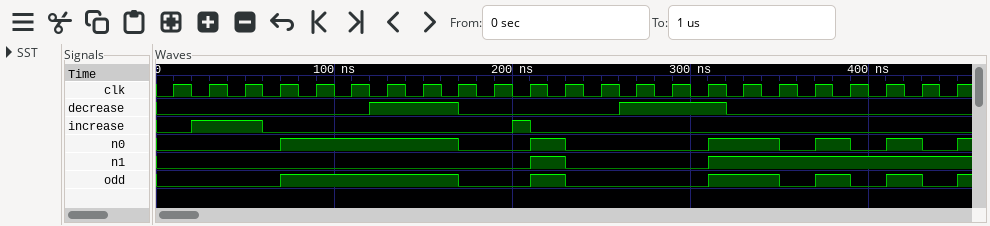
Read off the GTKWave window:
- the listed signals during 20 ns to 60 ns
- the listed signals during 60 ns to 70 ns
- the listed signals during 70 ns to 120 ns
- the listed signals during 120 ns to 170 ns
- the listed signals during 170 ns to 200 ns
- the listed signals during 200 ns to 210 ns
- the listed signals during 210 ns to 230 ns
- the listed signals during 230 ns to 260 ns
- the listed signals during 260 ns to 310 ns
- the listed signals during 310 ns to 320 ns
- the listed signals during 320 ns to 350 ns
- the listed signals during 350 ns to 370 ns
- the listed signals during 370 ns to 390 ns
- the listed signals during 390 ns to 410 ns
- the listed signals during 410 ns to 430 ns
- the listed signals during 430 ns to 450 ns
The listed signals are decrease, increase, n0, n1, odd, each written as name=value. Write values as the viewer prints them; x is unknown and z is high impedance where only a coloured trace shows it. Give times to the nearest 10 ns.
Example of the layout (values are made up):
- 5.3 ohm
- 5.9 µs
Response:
- decrease=0, increase=1, n0=0, n1=0, odd=0
- decrease=0, increase=0, n0=0, n1=0, odd=0
- decrease=0, increase=0, n0=1, n1=0, odd=1
- decrease=1, increase=0, n0=1, n1=0, odd=1
- decrease=0, increase=0, n0=0, n1=0, odd=0
- decrease=0, increase=1, n0=0, n1=0, odd=0
- decrease=0, increase=0, n0=1, n1=1, odd=1
- decrease=0, increase=0, n0=0, n1=0, odd=0
- decrease=1, increase=0, n0=0, n1=0, odd=0
- decrease=1, increase=0, n0=1, n1=1, odd=1
- decrease=0, increase=0, n0=1, n1=1, odd=1
- decrease=0, increase=0, n0=0, n1=1, odd=0
- decrease=0, increase=0, n0=1, n1=1, odd=1
- decrease=0, increase=0, n0=0, n1=1, odd=0
- decrease=0, increase=0, n0=1, n1=1, odd=1
- decrease=0, increase=0, n0=0, n1=1, odd=0
